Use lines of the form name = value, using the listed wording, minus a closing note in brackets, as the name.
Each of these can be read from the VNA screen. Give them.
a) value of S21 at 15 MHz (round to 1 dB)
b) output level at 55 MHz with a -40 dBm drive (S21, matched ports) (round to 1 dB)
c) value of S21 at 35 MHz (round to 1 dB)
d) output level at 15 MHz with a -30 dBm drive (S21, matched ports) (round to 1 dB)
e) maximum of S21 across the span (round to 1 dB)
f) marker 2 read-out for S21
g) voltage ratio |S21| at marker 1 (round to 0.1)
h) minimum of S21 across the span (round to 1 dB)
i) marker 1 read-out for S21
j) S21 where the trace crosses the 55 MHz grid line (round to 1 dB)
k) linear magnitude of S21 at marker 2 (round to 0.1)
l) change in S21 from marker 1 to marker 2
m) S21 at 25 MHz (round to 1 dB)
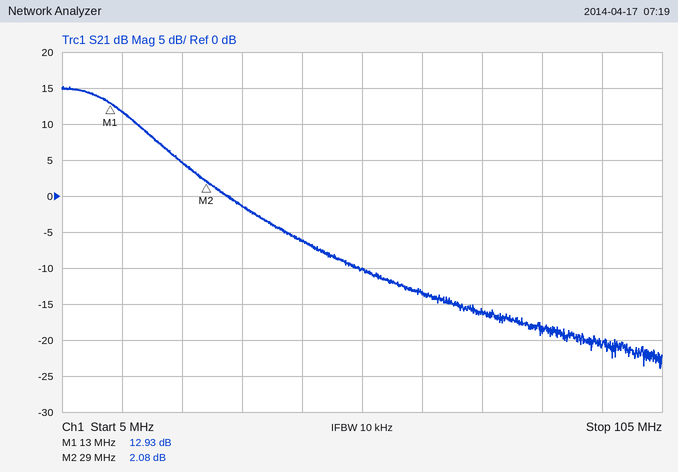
value of S21 at 15 MHz = 12 dB
output level at 55 MHz with a -40 dBm drive (S21, matched ports) = -50 dBm
value of S21 at 35 MHz = -1 dB
output level at 15 MHz with a -30 dBm drive (S21, matched ports) = -18 dBm
maximum of S21 across the span = 15 dB
marker 2 read-out for S21 = 2.08 dB
voltage ratio |S21| at marker 1 = 4.4
minimum of S21 across the span = -24 dB
marker 1 read-out for S21 = 12.93 dB
S21 where the trace crosses the 55 MHz grid line = -10 dB
linear magnitude of S21 at marker 2 = 1.3
change in S21 from marker 1 to marker 2 = -10.85 dB
S21 at 25 MHz = 5 dB
